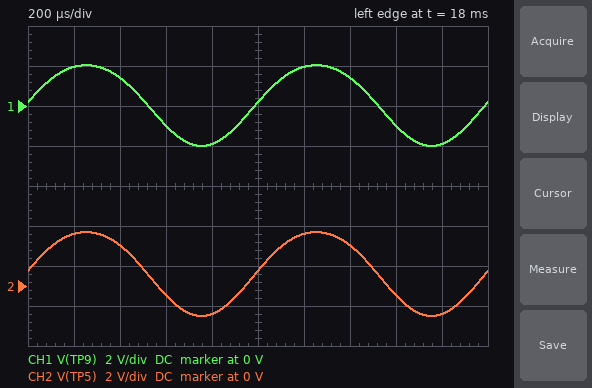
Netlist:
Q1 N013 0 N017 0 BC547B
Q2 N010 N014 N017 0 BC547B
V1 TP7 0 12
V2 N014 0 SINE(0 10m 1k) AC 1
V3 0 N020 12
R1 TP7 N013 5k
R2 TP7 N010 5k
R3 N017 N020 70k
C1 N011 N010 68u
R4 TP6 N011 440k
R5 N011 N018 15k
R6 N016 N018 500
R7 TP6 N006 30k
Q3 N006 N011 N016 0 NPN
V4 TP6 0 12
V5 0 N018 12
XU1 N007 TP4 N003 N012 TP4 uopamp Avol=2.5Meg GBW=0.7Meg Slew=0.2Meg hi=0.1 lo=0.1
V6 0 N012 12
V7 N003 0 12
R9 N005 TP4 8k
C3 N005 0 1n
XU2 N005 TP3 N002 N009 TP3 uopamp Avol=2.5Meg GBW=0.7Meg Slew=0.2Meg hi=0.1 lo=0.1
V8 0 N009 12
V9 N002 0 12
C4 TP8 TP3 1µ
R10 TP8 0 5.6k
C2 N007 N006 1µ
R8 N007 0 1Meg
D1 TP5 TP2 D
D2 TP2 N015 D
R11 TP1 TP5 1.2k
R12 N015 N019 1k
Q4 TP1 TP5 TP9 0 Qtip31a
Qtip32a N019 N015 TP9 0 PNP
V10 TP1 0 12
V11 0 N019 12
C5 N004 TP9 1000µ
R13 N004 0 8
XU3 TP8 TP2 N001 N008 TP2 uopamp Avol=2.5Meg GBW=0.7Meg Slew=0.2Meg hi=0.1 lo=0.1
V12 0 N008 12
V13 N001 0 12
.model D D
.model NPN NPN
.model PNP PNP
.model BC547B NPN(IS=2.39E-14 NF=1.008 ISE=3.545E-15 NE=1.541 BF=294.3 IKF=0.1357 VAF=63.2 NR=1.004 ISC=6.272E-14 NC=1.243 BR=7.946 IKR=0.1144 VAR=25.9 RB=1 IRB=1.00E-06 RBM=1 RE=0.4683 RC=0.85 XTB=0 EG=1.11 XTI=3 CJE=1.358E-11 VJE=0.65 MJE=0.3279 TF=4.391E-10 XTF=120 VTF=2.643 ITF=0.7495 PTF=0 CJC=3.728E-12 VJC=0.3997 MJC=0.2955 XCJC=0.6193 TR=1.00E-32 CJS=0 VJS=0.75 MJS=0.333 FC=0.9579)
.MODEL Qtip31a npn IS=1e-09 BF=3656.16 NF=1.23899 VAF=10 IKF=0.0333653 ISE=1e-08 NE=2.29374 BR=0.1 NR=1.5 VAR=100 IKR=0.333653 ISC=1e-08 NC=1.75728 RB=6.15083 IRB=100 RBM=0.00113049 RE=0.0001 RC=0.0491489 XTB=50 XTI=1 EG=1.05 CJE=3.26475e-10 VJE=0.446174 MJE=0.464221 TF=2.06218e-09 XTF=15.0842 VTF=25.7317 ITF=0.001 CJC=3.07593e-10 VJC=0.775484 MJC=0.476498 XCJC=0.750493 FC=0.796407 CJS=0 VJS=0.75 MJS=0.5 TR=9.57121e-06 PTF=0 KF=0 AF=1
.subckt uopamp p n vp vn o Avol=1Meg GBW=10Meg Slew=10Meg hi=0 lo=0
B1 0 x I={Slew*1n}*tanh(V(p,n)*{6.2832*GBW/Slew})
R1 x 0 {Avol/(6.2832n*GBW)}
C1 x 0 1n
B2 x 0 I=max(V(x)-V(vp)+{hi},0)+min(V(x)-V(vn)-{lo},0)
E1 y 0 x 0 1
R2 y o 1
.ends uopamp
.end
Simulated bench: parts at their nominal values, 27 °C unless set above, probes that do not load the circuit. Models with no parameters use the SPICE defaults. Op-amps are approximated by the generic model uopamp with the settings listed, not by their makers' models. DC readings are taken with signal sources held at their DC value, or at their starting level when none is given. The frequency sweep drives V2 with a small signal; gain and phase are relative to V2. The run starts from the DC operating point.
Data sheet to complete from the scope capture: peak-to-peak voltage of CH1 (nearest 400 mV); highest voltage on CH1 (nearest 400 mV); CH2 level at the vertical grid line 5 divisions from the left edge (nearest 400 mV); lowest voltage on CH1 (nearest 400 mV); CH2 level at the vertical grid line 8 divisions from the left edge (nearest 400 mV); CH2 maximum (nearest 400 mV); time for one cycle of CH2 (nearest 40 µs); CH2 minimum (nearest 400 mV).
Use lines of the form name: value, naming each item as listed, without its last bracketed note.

peak-to-peak voltage of CH1: 4.0 V
highest voltage on CH1: 2.0 V
CH2 level at the vertical grid line 5 divisions from the left edge: 800 mV
lowest voltage on CH1: -2.0 V
CH2 level at the vertical grid line 8 divisions from the left edge: -400 mV
CH2 maximum: 2.8 V
time for one cycle of CH2: 1.00 ms
CH2 minimum: -1.6 V
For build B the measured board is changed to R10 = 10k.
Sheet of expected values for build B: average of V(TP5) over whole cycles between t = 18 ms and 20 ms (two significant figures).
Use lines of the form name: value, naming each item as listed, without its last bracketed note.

average of V(TP5) over whole cycles between t = 18 ms and 20 ms: 690 mV
